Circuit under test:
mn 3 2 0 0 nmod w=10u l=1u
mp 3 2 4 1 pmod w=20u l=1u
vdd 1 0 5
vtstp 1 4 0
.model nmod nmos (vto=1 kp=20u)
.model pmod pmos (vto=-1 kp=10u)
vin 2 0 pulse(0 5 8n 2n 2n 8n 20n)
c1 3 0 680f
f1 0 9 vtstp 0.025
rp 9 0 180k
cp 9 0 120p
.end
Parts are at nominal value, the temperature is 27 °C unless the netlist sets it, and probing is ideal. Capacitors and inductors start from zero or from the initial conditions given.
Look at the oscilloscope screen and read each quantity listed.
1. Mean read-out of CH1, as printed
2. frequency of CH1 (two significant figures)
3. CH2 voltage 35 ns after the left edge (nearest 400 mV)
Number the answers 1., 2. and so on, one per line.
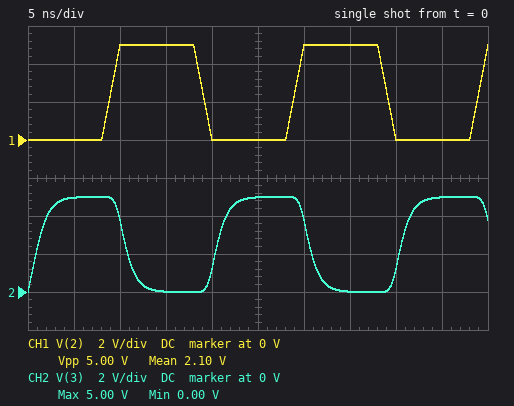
1. 2.10 V
2. 50 MHz
3. 0 V
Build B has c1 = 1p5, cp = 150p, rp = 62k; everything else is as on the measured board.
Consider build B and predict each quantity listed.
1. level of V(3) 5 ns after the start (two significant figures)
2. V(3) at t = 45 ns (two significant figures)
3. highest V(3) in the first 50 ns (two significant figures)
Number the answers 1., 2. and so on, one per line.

1. 4.2 V
2. 4.4 V
3. 4.9 V
